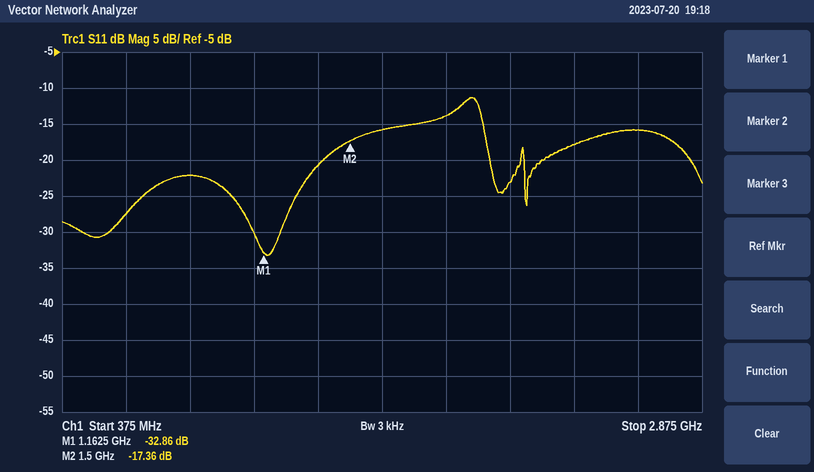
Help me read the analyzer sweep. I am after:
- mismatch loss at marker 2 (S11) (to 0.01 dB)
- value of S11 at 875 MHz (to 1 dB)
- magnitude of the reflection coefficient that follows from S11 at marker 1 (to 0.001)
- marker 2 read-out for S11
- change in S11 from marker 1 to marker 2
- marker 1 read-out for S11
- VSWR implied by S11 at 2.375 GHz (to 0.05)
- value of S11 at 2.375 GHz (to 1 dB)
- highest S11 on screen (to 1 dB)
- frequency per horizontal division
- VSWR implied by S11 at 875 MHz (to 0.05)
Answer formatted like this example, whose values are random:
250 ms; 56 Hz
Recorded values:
0.08 dB; -22 dB; 0.023; -17.36 dB; 15.50 dB; -32.86 dB; 1.30; -18 dB; -11 dB; 250 MHz; 1.15
